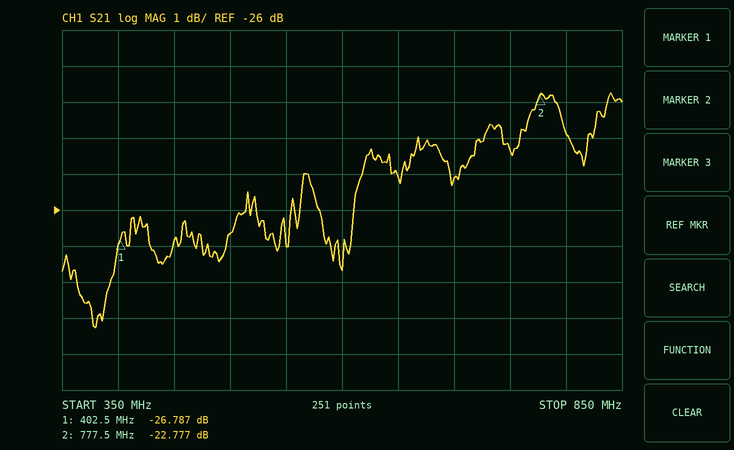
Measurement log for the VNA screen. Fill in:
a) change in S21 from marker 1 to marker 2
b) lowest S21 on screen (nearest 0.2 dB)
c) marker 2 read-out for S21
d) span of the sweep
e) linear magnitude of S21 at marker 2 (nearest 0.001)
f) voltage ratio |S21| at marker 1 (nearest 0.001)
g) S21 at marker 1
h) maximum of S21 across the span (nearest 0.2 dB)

4.010 dB
-29.2 dB
-22.777 dB
500 MHz
0.073
0.046
-26.787 dB
-22.8 dB
